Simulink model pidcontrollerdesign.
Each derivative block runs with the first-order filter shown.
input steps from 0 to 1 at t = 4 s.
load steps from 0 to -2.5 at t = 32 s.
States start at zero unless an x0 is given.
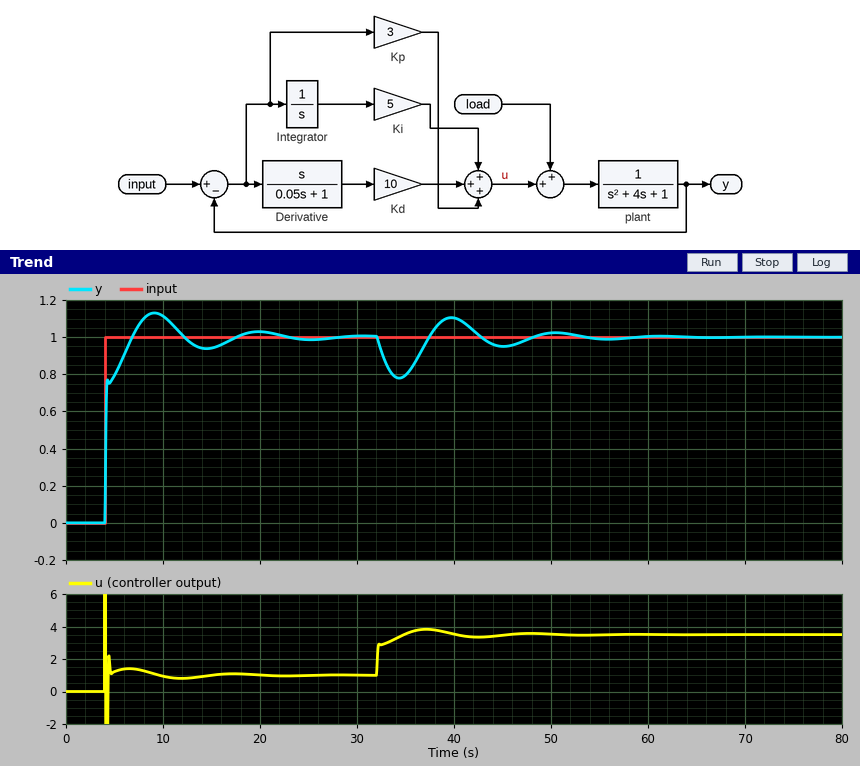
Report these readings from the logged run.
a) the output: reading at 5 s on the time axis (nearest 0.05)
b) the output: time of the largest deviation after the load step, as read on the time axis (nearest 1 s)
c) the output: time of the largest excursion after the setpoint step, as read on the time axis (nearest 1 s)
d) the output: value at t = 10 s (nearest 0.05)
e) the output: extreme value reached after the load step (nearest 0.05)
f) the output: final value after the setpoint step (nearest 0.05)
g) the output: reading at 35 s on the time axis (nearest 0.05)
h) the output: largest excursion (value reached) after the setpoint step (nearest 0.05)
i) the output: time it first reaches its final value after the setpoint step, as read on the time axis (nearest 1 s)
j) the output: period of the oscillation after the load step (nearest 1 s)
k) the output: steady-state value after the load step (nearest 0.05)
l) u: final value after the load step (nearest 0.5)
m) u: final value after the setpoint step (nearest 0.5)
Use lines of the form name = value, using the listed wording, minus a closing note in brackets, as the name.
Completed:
the output: reading at 5 s on the time axis = 0.80
the output: time of the largest deviation after the load step, as read on the time axis = 34 s
the output: time of the largest excursion after the setpoint step, as read on the time axis = 9 s
the output: value at t = 10 s = 1.10
the output: extreme value reached after the load step = 0.80
the output: final value after the setpoint step = 1.00
the output: reading at 35 s on the time axis = 0.80
the output: largest excursion (value reached) after the setpoint step = 1.15
the output: time it first reaches its final value after the setpoint step, as read on the time axis = 7 s
the output: period of the oscillation after the load step = 11 s
the output: steady-state value after the load step = 1.00
u: final value after the load step = 3.5
u: final value after the setpoint step = 1.0
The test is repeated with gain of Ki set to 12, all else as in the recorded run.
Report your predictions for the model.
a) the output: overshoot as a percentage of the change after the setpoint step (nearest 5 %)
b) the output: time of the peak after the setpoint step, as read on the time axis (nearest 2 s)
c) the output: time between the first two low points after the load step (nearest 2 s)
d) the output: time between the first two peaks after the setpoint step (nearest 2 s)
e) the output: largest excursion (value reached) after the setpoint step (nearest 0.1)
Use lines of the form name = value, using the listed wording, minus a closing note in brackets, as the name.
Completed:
the output: overshoot as a percentage of the change after the setpoint step = 20 %
the output: time of the peak after the setpoint step, as read on the time axis = 8 s
the output: time between the first two low points after the load step = 6 s
the output: time between the first two peaks after the setpoint step = 6 s
the output: largest excursion (value reached) after the setpoint step = 1.2
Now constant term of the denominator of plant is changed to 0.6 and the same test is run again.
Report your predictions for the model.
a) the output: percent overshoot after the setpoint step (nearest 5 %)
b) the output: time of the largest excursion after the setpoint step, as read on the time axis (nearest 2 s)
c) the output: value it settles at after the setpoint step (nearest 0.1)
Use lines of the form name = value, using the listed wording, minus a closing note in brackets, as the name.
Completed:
the output: percent overshoot after the setpoint step = 15 %
the output: time of the largest excursion after the setpoint step, as read on the time axis = 8 s
the output: value it settles at after the setpoint step = 1.0
